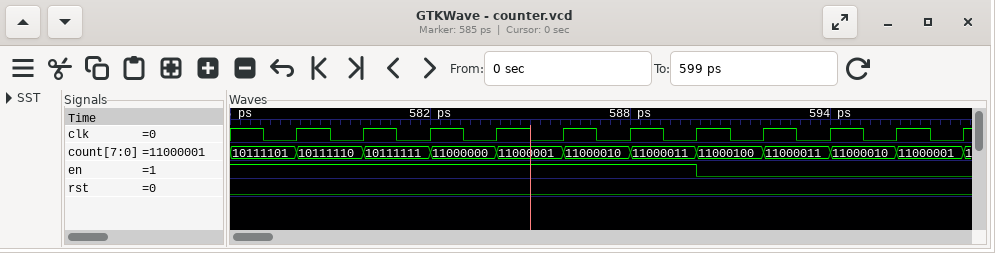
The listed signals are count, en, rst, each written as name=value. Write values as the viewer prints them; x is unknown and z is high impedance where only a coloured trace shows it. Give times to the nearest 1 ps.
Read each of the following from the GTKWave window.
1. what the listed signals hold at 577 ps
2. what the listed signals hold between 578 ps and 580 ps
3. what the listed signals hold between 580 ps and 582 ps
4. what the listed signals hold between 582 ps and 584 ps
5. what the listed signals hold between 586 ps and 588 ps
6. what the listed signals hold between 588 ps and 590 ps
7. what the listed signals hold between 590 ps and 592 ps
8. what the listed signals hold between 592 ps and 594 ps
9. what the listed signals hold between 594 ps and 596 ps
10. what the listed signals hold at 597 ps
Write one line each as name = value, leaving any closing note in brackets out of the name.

what the listed signals hold at 577 ps = count=10111101, en=1, rst=0
what the listed signals hold between 578 ps and 580 ps = count=10111110, en=1, rst=0
what the listed signals hold between 580 ps and 582 ps = count=10111111, en=1, rst=0
what the listed signals hold between 582 ps and 584 ps = count=11000000, en=1, rst=0
what the listed signals hold between 586 ps and 588 ps = count=11000010, en=1, rst=0
what the listed signals hold between 588 ps and 590 ps = count=11000011, en=1, rst=0
what the listed signals hold between 590 ps and 592 ps = count=11000100, en=0, rst=0
what the listed signals hold between 592 ps and 594 ps = count=11000011, en=0, rst=0
what the listed signals hold between 594 ps and 596 ps = count=11000010, en=0, rst=0
what the listed signals hold at 597 ps = count=11000001, en=0, rst=0
